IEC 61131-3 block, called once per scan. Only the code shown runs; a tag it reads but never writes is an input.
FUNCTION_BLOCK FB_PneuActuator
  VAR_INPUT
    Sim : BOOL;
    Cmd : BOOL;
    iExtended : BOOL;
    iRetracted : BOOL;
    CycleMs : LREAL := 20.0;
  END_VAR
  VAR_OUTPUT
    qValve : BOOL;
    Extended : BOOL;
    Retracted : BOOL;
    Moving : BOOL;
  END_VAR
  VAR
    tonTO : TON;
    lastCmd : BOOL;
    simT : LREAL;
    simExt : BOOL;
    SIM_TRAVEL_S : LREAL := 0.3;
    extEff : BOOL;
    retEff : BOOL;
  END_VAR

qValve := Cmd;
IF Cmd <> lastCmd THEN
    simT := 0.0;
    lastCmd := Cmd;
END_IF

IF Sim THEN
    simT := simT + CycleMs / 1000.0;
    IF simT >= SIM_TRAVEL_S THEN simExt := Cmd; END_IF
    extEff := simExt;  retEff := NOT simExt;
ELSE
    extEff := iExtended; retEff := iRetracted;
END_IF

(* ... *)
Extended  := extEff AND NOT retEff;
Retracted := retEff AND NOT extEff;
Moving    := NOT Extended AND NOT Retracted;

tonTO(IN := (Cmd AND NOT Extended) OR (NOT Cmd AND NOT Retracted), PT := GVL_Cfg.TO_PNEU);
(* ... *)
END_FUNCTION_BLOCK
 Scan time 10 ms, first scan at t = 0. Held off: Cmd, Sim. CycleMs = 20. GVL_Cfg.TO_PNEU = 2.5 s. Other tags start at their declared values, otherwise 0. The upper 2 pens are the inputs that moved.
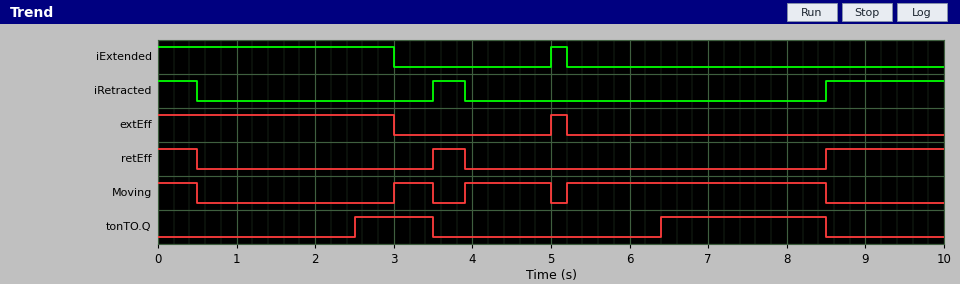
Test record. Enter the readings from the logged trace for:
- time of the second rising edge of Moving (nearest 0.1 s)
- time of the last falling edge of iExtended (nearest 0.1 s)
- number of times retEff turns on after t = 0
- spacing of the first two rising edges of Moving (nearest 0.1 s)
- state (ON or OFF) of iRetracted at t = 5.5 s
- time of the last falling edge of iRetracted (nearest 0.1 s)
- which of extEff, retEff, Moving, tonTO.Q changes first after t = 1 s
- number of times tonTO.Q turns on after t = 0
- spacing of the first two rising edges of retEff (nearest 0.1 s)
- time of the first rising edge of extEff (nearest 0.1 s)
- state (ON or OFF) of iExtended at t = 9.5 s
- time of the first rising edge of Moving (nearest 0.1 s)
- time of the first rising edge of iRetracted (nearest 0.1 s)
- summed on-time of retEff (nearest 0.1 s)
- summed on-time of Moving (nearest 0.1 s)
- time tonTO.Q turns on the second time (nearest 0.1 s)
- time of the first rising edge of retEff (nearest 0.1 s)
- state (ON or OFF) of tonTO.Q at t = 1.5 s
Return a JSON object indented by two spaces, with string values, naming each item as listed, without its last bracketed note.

{
  "time of the second rising edge of Moving": "3.9 s",
  "time of the last falling edge of iExtended": "5.2 s",
  "number of times retEff turns on after t = 0": "2",
  "spacing of the first two rising edges of Moving": "0.9 s",
  "state (ON or OFF) of iRetracted at t = 5.5 s": "OFF",
  "time of the last falling edge of iRetracted": "3.9 s",
  "which of extEff, retEff, Moving, tonTO.Q changes first after t = 1 s": "tonTO.Q",
  "number of times tonTO.Q turns on after t = 0": "2",
  "spacing of the first two rising edges of retEff": "5.0 s",
  "time of the first rising edge of extEff": "5.0 s",
  "state (ON or OFF) of iExtended at t = 9.5 s": "OFF",
  "time of the first rising edge of Moving": "3.0 s",
  "time of the first rising edge of iRetracted": "3.5 s",
  "summed on-time of retEff": "2.4 s",
  "summed on-time of Moving": "5.4 s",
  "time tonTO.Q turns on the second time": "6.4 s",
  "time of the first rising edge of retEff": "3.5 s",
  "state (ON or OFF) of tonTO.Q at t = 1.5 s": "OFF"
}
